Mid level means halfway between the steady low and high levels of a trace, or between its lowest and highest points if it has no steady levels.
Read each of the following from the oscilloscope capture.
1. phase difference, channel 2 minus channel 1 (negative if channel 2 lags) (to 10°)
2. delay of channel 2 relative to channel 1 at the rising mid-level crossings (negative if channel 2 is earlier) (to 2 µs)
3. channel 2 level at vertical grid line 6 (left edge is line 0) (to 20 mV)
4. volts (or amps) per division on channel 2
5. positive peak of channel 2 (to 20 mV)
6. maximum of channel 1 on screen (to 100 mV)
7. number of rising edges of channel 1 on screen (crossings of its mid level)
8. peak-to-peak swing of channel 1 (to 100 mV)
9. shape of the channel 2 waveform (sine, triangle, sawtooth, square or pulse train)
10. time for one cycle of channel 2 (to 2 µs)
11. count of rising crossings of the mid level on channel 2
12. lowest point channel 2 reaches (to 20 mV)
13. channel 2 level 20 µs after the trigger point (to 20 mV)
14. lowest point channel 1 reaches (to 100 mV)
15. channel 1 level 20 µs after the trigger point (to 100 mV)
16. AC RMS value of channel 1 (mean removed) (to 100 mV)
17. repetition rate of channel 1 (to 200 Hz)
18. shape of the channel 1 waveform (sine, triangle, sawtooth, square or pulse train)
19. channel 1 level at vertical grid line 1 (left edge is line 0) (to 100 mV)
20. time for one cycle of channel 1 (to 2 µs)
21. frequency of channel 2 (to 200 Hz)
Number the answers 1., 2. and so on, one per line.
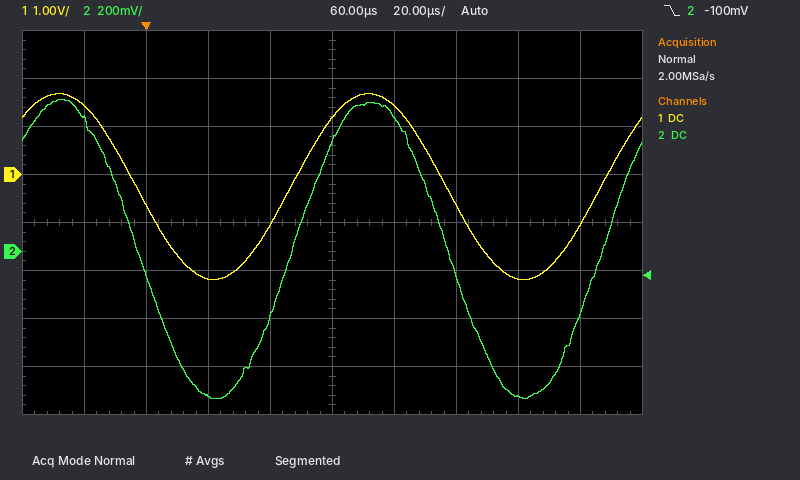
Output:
1. 0°
2. 0 µs
3. 560 mV
4. 200 mV
5. 640 mV
6. 1.7 V
7. 2
8. 3.9 V
9. sine
10. 100 µs
11. 2
12. -620 mV
13. -600 mV
14. -2.2 V
15. -2.2 V
16. 1.4 V
17. 10.0 kHz
18. sine
19. 1.4 V
20. 100 µs
21. 10.0 kHz
